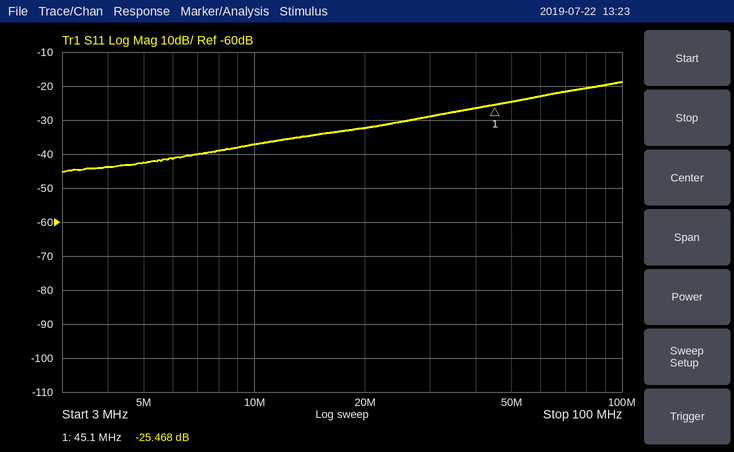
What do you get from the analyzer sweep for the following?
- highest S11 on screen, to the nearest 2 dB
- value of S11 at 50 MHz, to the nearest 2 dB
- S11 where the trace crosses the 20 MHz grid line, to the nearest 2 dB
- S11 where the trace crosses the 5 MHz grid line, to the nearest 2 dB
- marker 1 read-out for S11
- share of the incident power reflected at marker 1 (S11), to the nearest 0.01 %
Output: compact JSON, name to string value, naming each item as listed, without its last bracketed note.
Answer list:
{"highest S11 on screen, to the nearest 2 dB": "-18 dB", "value of S11 at 50 MHz, to the nearest 2 dB": "-24 dB", "S11 where the trace crosses the 20 MHz grid line, to the nearest 2 dB": "-32 dB", "S11 where the trace crosses the 5 MHz grid line, to the nearest 2 dB": "-42 dB", "marker 1 read-out for S11": "-25.468 dB", "share of the incident power reflected at marker 1 (S11), to the nearest 0.01 %": "0.28 %"}
